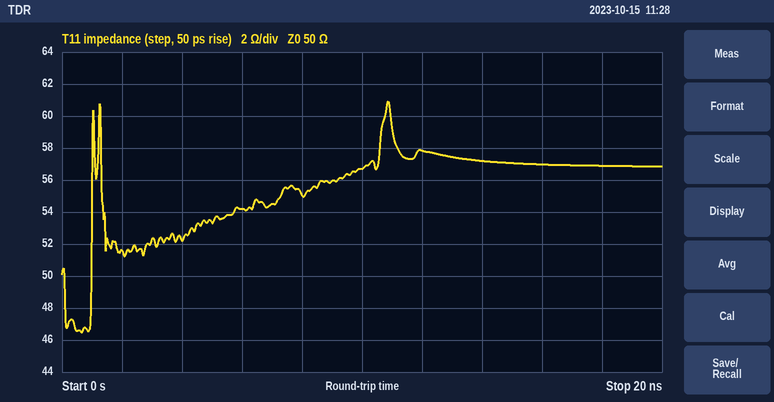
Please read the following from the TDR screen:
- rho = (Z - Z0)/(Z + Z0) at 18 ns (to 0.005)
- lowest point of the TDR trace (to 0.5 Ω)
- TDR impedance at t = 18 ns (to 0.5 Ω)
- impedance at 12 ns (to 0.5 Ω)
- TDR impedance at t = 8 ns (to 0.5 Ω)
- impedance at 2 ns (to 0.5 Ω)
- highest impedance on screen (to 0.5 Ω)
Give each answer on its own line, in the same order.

+0.065
46.5 Ω
57.0 Ω
58.0 Ω
55.0 Ω
51.5 Ω
61.0 Ω
